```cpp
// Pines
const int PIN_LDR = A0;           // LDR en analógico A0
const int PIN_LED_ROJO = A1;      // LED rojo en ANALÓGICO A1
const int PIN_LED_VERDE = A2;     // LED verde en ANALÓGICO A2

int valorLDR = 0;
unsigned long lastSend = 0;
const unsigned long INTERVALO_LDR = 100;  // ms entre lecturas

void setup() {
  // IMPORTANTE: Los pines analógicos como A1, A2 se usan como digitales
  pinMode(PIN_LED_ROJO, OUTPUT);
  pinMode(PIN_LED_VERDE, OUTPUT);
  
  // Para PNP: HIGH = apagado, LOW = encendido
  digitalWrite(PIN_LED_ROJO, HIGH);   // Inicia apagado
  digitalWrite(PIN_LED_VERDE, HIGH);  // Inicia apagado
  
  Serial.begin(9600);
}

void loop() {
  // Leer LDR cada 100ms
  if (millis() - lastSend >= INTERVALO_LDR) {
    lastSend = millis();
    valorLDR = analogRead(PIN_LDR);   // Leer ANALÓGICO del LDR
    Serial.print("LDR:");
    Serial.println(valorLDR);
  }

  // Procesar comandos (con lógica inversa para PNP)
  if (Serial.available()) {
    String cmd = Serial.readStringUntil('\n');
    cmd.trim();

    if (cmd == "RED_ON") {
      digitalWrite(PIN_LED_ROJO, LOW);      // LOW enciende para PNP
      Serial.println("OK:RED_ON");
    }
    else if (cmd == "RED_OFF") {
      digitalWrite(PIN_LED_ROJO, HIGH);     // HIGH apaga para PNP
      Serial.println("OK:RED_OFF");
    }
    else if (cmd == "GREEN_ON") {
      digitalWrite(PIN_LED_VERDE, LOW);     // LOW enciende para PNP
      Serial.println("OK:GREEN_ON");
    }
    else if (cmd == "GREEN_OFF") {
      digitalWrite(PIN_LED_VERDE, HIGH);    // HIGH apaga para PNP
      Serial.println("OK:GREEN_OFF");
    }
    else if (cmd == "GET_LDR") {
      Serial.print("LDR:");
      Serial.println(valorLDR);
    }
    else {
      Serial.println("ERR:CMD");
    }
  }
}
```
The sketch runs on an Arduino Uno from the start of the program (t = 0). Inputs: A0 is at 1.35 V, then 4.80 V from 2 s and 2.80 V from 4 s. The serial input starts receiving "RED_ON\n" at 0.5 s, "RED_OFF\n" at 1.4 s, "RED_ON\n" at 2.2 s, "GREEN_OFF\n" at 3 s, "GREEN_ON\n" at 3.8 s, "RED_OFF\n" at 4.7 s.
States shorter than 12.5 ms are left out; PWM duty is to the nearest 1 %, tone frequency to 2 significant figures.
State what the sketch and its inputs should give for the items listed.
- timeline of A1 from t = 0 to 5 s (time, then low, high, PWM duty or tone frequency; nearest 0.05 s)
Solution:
0 s high; 0.5 s low; 1.4 s high; 2.2 s low; 4.7 s high
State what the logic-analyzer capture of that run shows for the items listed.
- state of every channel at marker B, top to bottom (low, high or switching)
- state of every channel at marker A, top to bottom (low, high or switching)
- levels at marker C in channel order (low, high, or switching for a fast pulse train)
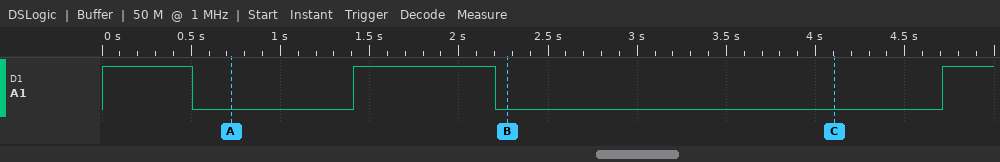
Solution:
A1 low
A1 low
A1 low
